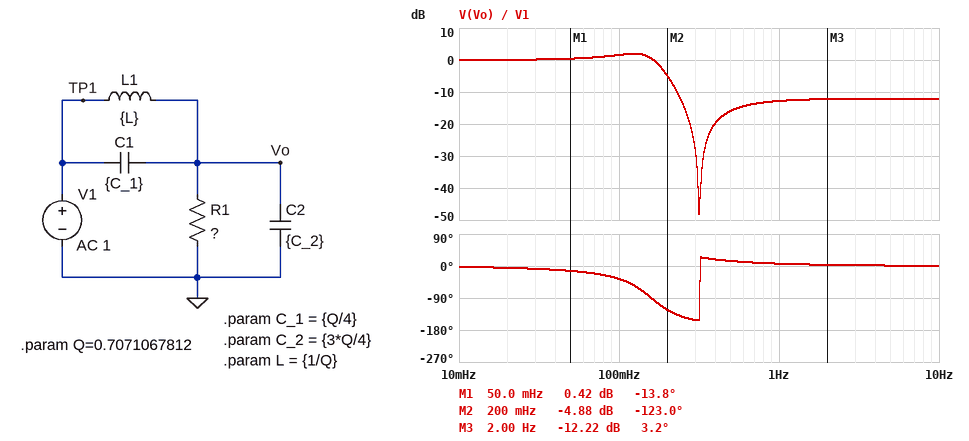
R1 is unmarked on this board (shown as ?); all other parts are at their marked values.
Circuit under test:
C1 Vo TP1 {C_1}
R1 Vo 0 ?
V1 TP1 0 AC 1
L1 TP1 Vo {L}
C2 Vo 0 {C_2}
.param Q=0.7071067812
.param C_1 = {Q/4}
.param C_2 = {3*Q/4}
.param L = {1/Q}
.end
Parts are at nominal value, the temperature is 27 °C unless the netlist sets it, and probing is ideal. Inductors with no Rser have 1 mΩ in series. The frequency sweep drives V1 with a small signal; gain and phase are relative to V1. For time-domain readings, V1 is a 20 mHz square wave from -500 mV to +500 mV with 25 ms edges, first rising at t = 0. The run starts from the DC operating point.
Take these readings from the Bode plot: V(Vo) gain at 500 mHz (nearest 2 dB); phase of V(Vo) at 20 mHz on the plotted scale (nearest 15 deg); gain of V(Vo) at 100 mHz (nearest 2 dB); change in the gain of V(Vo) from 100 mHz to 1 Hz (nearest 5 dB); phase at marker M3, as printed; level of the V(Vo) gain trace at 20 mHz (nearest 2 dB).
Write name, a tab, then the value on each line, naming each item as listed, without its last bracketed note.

V(Vo) gain at 500 mHz	-16 dB
phase of V(Vo) at 20 mHz on the plotted scale	0 deg
gain of V(Vo) at 100 mHz	2 dB
change in the gain of V(Vo) from 100 mHz to 1 Hz	-15 dB
phase at marker M3, as printed	3.2 deg
level of the V(Vo) gain trace at 20 mHz	0 dB
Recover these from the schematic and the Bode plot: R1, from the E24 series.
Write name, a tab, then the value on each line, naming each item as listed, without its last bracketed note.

R1, from the E24 series	2 Ω
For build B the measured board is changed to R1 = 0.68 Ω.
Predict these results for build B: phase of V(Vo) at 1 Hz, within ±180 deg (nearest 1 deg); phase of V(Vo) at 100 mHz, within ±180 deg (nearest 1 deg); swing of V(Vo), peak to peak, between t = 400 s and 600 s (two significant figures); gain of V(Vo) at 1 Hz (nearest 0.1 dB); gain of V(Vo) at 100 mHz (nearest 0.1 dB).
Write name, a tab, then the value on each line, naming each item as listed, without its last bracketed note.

phase of V(Vo) at 1 Hz, within ±180 deg	19 deg
phase of V(Vo) at 100 mHz, within ±180 deg	-65 deg
swing of V(Vo), peak to peak, between t = 400 s and 600 s	1.0 V
gain of V(Vo) at 1 Hz	-13.2 dB
gain of V(Vo) at 100 mHz	-4.1 dB
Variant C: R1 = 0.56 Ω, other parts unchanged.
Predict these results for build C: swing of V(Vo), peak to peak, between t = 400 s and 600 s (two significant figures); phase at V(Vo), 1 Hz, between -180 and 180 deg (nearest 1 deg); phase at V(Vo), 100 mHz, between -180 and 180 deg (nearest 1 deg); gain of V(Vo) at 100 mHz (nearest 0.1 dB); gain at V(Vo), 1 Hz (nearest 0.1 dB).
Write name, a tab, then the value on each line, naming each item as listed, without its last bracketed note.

swing of V(Vo), peak to peak, between t = 400 s and 600 s	1.0 V
phase at V(Vo), 1 Hz, between -180 and 180 deg	22 deg
phase at V(Vo), 100 mHz, between -180 and 180 deg	-69 deg
gain of V(Vo) at 100 mHz	-5.5 dB
gain at V(Vo), 1 Hz	-13.4 dB
